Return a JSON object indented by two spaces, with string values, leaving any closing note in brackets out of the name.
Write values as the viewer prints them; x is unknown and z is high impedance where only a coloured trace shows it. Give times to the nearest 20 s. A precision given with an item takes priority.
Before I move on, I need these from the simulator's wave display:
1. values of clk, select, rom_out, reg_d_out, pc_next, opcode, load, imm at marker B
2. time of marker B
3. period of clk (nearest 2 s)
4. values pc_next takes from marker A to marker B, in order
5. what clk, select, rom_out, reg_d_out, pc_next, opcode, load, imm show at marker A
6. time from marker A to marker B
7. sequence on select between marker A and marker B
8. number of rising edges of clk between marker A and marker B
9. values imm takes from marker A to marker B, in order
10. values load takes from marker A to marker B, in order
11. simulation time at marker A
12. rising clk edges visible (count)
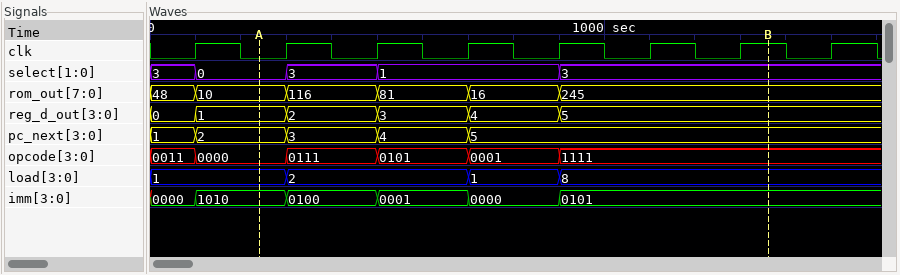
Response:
{
  "values of clk, select, rom_out, reg_d_out, pc_next, opcode, load, imm at marker B": "clk=1, select=3, rom_out=245, reg_d_out=5, pc_next=5, opcode=1111, load=8, imm=0101",
  "time of marker B": "1360 s",
  "period of clk": "200 s",
  "values pc_next takes from marker A to marker B, in order": "2, 3, 4, 5",
  "what clk, select, rom_out, reg_d_out, pc_next, opcode, load, imm show at marker A": "clk=0, select=0, rom_out=10, reg_d_out=1, pc_next=2, opcode=0000, load=1, imm=1010",
  "time from marker A to marker B": "1120 s",
  "sequence on select between marker A and marker B": "0, 3, 1, 3",
  "number of rising edges of clk between marker A and marker B": "6",
  "values imm takes from marker A to marker B, in order": "1010, 0100, 0001, 0000, 0101",
  "values load takes from marker A to marker B, in order": "1, 2, 1, 8",
  "simulation time at marker A": "240 s",
  "rising clk edges visible": "8"
}
